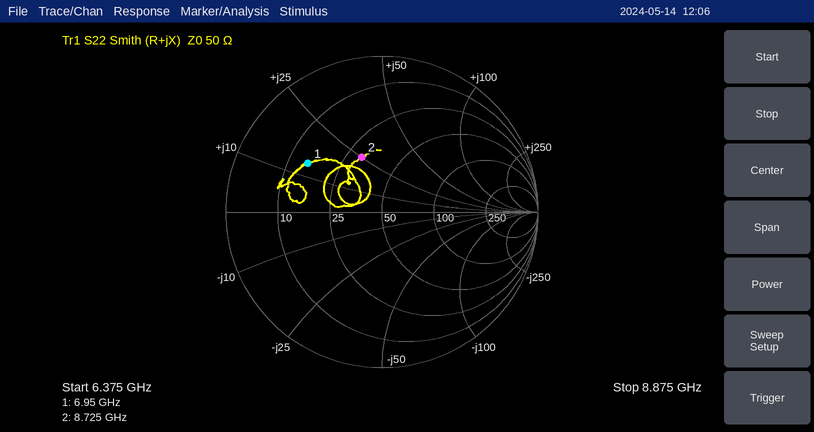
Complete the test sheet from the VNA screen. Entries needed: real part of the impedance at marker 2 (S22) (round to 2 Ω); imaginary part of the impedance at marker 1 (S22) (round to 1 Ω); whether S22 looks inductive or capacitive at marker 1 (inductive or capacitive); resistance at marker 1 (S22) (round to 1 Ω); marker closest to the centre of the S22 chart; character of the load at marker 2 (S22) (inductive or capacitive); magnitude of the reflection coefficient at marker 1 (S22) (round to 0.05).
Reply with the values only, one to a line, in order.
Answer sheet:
30 Ω
+14 Ω
inductive
15 Ω
marker 2
inductive
0.55
